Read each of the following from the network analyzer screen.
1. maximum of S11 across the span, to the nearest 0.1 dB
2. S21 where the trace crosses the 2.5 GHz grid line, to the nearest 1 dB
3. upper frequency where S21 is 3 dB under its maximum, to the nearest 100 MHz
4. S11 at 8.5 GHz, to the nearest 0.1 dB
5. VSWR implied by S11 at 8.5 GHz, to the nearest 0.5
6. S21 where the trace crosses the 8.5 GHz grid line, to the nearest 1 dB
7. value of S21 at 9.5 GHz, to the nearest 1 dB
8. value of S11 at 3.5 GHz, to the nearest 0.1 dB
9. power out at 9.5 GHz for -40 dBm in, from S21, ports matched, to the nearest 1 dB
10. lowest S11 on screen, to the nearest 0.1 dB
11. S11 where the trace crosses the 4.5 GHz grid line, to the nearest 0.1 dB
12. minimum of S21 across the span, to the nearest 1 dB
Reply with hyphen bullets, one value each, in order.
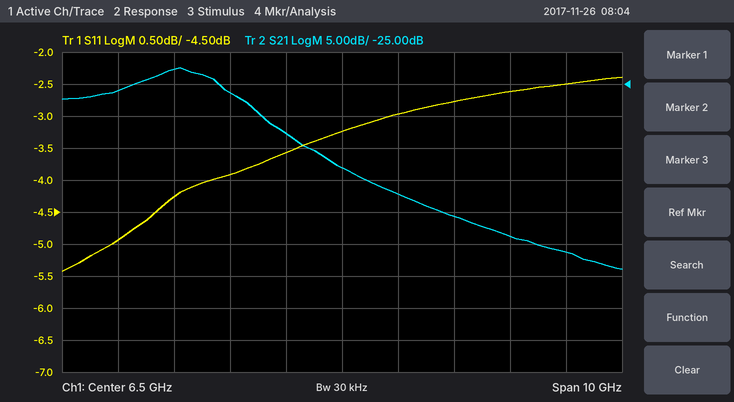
- -2.4 dB
- -26 dB
- 4.4 GHz
- -2.8 dB
- 6.5
- -46 dB
- -49 dB
- -4.3 dB
- -89 dBm
- -5.4 dB
- -3.9 dB
- -54 dB
